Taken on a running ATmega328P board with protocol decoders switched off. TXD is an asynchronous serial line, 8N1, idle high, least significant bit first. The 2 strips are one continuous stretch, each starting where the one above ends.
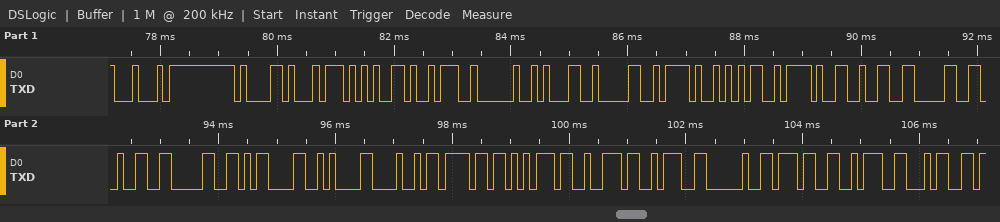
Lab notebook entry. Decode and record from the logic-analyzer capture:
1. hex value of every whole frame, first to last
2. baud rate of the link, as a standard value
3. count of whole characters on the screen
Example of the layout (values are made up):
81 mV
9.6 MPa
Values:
44 61 74 65 3A 20 31 30 2F 35 2F 32 30 32 30 0D 0A 48 6F 75 72 3A 20 37 3A 34
9600 baud
26
